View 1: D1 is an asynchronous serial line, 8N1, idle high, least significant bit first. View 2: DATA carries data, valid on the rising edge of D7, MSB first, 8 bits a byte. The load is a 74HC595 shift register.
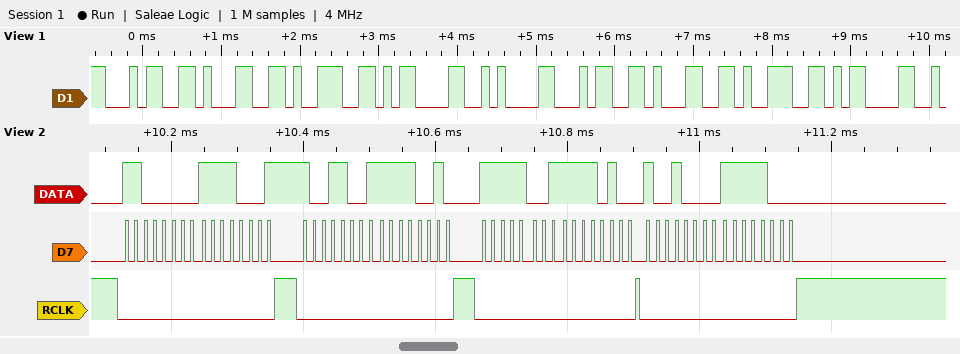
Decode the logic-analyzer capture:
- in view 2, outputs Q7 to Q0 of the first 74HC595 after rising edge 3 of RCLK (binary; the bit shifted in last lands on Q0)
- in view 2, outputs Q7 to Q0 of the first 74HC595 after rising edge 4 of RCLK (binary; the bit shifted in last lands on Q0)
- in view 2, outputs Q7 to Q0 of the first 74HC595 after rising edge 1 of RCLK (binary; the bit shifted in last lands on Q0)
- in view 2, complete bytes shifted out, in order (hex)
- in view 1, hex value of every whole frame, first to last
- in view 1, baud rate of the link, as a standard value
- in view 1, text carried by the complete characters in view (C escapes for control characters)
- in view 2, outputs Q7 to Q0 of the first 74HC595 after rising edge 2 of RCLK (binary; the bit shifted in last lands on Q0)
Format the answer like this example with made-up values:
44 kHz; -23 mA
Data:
11110100; 11111000; 11110001; C0 F1 99 F2 F9 F4 90 F8; 34 31 39 0D 0A 34 31 39 0D; 9600 baud; "419\r\n419\r"; 11110010
